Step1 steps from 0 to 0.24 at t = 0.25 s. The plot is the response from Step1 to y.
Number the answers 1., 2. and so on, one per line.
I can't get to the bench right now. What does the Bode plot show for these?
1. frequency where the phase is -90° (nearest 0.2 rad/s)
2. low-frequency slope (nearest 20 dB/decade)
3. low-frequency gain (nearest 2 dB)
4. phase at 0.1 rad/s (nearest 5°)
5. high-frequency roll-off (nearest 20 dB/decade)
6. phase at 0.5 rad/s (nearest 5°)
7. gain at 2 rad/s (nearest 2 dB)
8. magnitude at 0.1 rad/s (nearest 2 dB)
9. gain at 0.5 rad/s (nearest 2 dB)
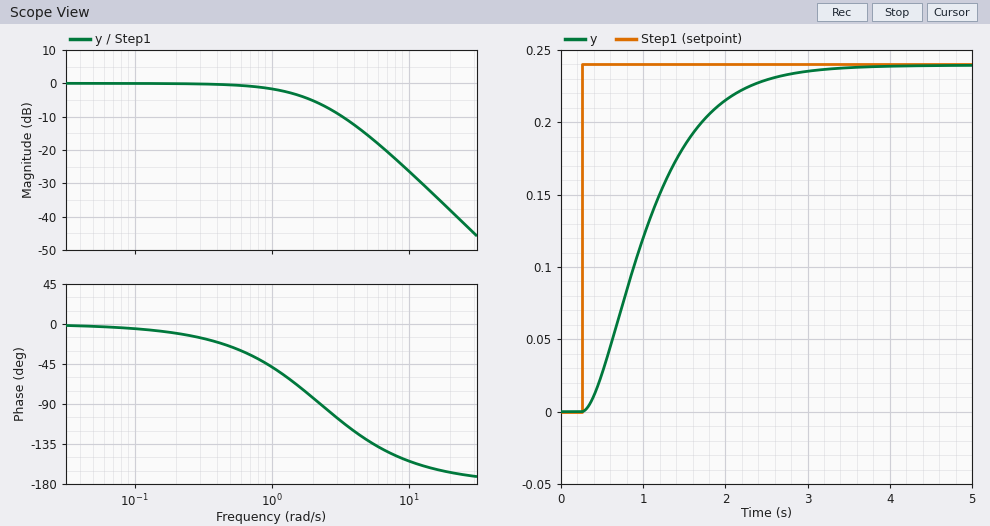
1. 2.2 rad/s
2. 0 dB/decade
3. 0 dB
4. -5°
5. -40 dB/decade
6. -25°
7. -6 dB
8. 0 dB
9. 0 dB
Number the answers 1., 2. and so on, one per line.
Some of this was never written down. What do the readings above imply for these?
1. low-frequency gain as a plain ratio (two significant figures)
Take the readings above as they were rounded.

1. 1.0
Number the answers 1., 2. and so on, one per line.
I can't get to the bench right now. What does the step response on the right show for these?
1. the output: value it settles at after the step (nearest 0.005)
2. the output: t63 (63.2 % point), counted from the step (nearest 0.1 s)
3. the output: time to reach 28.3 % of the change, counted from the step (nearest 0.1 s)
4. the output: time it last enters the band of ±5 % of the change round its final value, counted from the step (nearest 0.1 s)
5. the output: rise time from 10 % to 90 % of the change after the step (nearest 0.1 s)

1. 0.240
2. 1.0 s
3. 0.5 s
4. 2.2 s
5. 1.5 s
